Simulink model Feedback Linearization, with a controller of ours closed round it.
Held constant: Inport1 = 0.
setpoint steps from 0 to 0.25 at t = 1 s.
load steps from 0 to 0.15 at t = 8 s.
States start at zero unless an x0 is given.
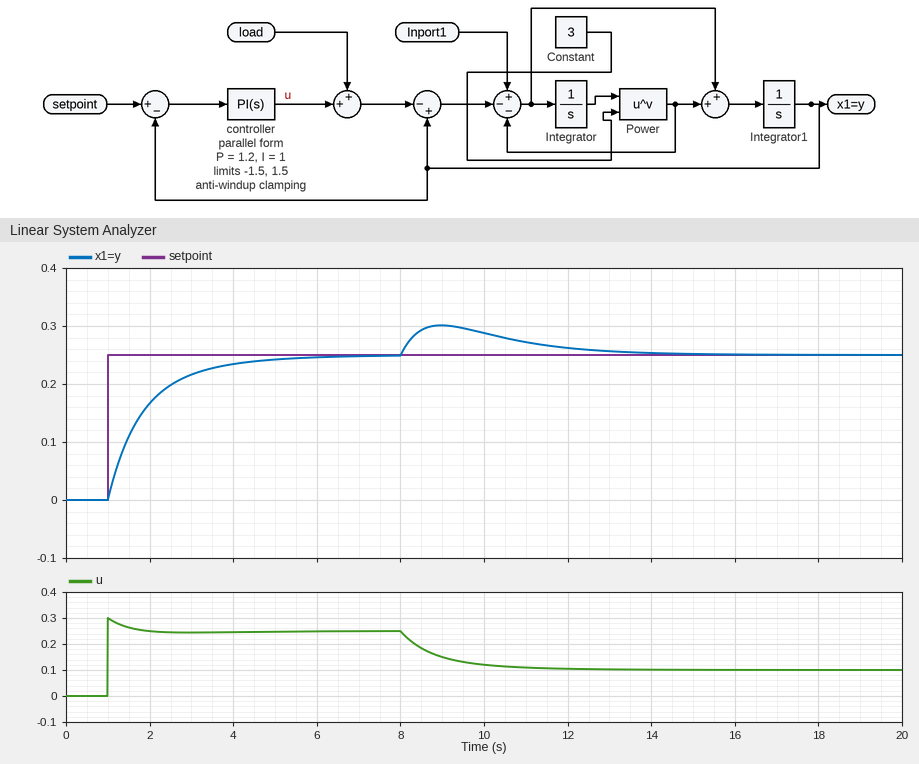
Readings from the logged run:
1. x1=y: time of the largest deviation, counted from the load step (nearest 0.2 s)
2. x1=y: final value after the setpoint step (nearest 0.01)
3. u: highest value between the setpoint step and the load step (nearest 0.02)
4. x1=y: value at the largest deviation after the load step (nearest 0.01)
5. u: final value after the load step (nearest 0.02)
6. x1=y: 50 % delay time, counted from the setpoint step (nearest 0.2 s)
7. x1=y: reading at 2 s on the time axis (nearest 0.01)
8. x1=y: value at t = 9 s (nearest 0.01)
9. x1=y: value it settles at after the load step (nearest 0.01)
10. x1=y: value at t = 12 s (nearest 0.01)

1.0 s
0.25
0.30
0.30
0.10
0.6 s
0.17
0.30
0.25
0.26
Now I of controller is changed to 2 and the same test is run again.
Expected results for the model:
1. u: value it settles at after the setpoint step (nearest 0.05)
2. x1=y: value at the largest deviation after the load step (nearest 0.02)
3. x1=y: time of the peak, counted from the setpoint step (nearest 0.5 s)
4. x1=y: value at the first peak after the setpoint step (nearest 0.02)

0.25
0.30
2.5 s
0.26
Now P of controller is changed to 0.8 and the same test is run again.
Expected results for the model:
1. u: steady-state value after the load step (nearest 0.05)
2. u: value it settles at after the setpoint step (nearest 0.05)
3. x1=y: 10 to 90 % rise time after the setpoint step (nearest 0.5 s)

0.10
0.25
2.0 s
